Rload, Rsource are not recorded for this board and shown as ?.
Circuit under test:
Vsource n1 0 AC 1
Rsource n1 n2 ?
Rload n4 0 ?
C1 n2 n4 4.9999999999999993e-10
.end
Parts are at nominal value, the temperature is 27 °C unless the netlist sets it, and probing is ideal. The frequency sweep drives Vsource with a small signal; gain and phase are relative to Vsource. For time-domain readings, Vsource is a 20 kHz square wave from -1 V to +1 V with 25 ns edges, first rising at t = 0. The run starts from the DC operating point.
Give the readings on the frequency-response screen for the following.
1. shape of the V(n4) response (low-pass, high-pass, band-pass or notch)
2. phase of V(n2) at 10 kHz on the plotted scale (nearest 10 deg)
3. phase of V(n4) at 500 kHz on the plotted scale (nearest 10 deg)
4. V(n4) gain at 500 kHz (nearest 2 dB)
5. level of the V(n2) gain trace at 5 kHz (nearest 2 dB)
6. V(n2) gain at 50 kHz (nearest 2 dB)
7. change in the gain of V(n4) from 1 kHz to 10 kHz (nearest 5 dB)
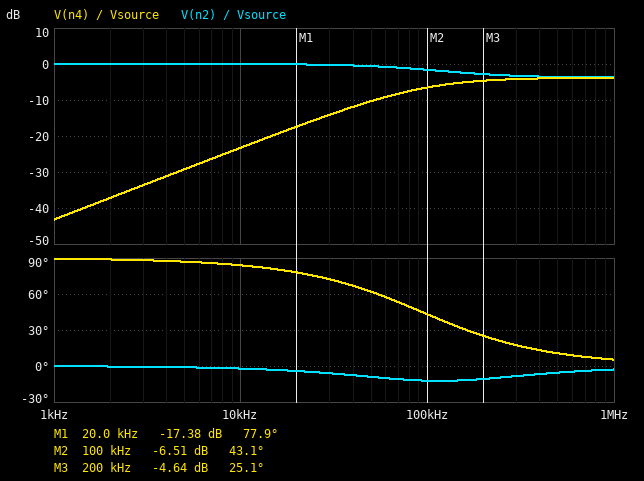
high-pass
0 deg
10 deg
-4 dB
0 dB
0 dB
20 dB
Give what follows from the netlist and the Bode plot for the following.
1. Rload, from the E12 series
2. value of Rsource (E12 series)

2.2 kΩ
1.2 kΩ
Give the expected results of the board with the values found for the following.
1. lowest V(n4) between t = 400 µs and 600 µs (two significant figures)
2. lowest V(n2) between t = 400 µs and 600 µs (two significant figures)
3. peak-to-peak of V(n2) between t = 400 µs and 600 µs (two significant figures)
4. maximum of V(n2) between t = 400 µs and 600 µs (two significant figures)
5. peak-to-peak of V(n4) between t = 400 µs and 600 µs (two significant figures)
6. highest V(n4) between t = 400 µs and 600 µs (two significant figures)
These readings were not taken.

-1.3 V
-1.0 V
2.0 V
1.0 V
2.6 V
1.3 V
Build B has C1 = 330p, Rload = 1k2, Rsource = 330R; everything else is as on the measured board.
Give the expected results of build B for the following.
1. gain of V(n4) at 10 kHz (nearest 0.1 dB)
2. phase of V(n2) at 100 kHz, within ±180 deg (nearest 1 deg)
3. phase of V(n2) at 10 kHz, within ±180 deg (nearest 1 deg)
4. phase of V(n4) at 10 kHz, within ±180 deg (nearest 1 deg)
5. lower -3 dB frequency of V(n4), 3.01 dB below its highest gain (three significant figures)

-32.1 dB
-4 deg
0 deg
88 deg
315 kHz
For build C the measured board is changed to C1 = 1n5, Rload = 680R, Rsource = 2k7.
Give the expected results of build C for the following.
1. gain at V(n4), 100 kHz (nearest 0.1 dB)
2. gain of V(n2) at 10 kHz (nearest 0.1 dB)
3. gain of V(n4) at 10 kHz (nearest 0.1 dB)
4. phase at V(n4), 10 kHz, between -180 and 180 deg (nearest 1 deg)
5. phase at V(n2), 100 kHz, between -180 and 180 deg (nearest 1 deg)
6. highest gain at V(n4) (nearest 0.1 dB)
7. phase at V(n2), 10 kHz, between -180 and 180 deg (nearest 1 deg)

-14.3 dB
-0.4 dB
-24.3 dB
72 deg
-40 deg
-13.9 dB
-14 deg
